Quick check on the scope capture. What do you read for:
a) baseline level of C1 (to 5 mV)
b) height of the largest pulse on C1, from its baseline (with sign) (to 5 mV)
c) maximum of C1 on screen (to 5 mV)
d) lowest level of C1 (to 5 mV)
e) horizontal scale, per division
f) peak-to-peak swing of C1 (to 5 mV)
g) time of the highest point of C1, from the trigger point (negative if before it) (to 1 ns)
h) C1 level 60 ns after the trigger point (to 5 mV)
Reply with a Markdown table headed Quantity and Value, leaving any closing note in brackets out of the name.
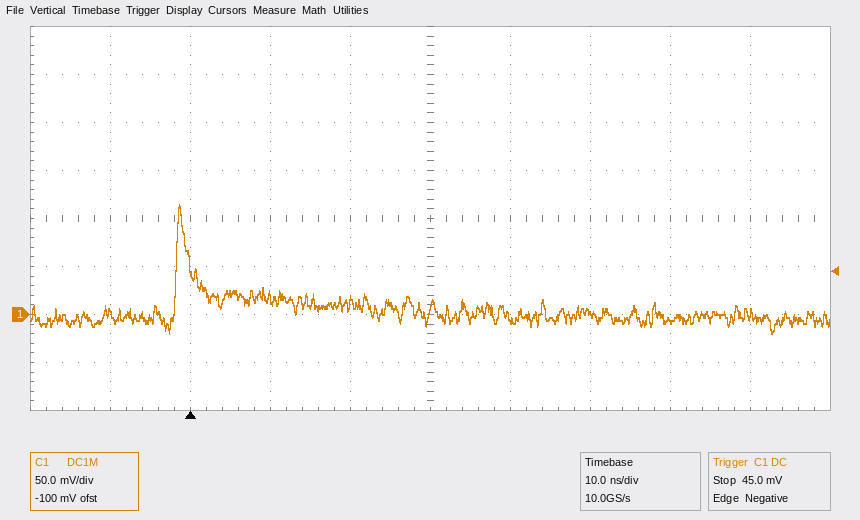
| Quantity | Value |
|---|---|
| baseline level of C1 | 0 mV |
| height of the largest pulse on C1, from its baseline (with sign) | +115 mV |
| maximum of C1 on screen | 115 mV |
| lowest level of C1 | -20 mV |
| horizontal scale, per division | 10 ns |
| peak-to-peak swing of C1 | 135 mV |
| time of the highest point of C1, from the trigger point (negative if before it) | -1 ns |
| C1 level 60 ns after the trigger point | -5 mV |
